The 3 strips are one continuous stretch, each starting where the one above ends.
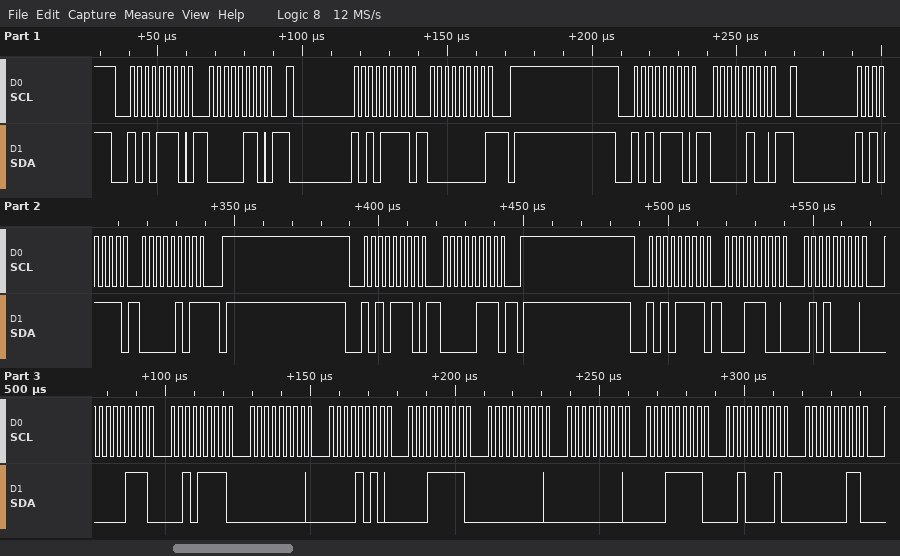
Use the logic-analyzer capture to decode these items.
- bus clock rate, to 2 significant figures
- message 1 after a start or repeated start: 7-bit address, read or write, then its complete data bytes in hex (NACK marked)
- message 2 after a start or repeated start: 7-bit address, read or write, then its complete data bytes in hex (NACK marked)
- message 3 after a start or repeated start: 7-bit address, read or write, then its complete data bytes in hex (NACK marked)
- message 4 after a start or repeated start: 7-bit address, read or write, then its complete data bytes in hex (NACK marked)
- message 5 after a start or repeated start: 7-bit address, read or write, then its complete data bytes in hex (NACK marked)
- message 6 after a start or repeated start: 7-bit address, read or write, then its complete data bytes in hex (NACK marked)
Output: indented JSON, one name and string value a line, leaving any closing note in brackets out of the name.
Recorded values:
{
  "bus clock rate, to 2 significant figures": "400 kHz",
  "message 1 after a start or repeated start: 7-bit address, read or write, then its complete data bytes in hex": "0x57 write: 06",
  "message 2 after a start or repeated start: 7-bit address, read or write, then its complete data bytes in hex": "0x57 read: 00 NACK",
  "message 3 after a start or repeated start: 7-bit address, read or write, then its complete data bytes in hex": "0x57 write: 04",
  "message 4 after a start or repeated start: 7-bit address, read or write, then its complete data bytes in hex": "0x57 read: 05 NACK",
  "message 5 after a start or repeated start: 7-bit address, read or write, then its complete data bytes in hex": "0x57 write: 07",
  "message 6 after a start or repeated start: 7-bit address, read or write, then its complete data bytes in hex": "0x57 read: 1C 50 07 2F 00 0A 1F 00 00 1F 21 03"
}
